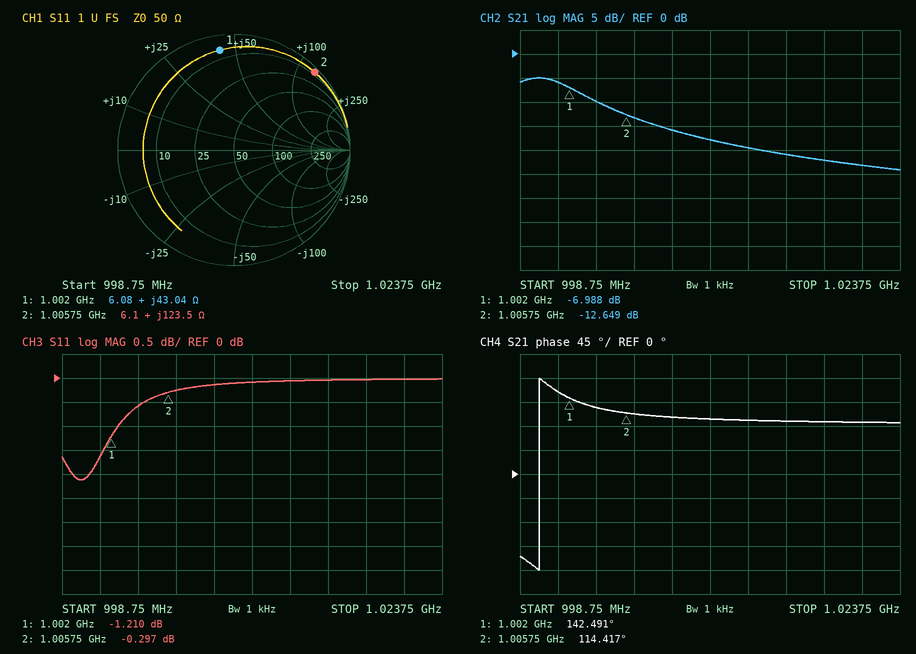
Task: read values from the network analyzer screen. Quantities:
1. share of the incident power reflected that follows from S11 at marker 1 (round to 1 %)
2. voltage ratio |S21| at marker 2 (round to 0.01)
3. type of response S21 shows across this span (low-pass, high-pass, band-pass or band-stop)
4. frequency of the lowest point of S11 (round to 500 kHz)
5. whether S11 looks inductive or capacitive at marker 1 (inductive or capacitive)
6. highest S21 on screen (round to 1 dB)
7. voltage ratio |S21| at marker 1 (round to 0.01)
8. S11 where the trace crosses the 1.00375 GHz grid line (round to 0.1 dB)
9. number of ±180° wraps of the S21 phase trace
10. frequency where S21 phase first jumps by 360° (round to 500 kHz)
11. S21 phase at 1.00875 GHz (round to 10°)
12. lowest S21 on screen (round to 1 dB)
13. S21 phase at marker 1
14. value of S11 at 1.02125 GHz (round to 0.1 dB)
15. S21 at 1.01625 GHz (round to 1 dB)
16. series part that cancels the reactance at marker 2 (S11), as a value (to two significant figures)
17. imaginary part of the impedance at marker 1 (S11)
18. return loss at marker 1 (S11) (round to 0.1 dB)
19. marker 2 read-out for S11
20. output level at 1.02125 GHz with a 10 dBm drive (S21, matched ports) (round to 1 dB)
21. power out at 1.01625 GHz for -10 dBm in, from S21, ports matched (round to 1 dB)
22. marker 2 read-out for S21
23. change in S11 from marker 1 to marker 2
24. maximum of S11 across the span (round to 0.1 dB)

76 %
0.23
low-pass
1.0000 GHz
inductive
-5 dB
0.45
-0.6 dB
1
1.0000 GHz
110°
-24 dB
142.491°
0.0 dB
-21 dB
1.3 pF
+43.04 Ω
1.2 dB
-0.297 dB
-13 dBm
-31 dBm
-12.649 dB
0.913 dB
0.0 dB
